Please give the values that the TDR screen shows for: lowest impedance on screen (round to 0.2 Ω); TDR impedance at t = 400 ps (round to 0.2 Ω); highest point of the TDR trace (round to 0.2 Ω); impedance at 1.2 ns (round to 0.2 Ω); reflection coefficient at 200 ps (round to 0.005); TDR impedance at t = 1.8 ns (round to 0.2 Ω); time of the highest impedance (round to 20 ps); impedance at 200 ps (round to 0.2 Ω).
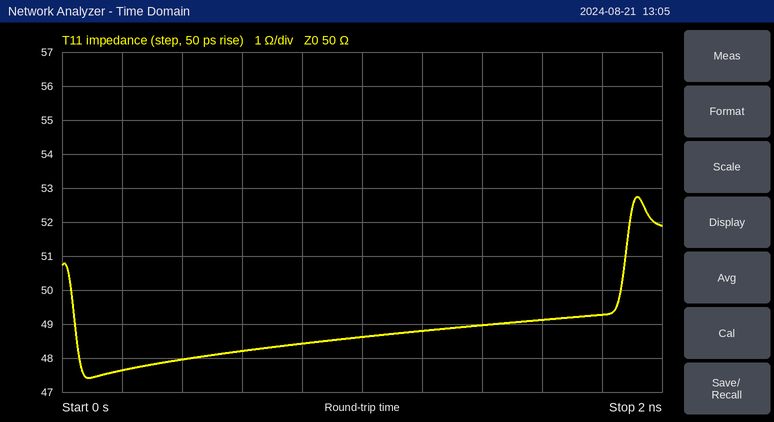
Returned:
47.4 Ω
48.0 Ω
52.8 Ω
48.8 Ω
-0.025
49.2 Ω
1.92 ns
47.6 Ω
